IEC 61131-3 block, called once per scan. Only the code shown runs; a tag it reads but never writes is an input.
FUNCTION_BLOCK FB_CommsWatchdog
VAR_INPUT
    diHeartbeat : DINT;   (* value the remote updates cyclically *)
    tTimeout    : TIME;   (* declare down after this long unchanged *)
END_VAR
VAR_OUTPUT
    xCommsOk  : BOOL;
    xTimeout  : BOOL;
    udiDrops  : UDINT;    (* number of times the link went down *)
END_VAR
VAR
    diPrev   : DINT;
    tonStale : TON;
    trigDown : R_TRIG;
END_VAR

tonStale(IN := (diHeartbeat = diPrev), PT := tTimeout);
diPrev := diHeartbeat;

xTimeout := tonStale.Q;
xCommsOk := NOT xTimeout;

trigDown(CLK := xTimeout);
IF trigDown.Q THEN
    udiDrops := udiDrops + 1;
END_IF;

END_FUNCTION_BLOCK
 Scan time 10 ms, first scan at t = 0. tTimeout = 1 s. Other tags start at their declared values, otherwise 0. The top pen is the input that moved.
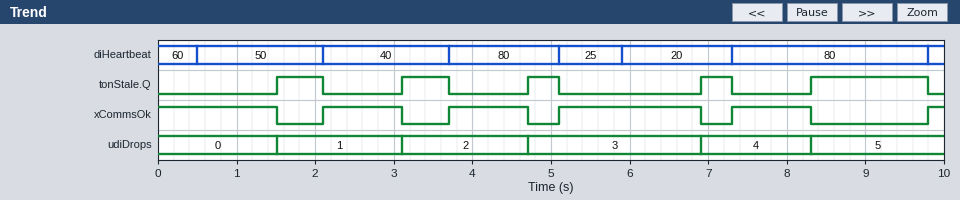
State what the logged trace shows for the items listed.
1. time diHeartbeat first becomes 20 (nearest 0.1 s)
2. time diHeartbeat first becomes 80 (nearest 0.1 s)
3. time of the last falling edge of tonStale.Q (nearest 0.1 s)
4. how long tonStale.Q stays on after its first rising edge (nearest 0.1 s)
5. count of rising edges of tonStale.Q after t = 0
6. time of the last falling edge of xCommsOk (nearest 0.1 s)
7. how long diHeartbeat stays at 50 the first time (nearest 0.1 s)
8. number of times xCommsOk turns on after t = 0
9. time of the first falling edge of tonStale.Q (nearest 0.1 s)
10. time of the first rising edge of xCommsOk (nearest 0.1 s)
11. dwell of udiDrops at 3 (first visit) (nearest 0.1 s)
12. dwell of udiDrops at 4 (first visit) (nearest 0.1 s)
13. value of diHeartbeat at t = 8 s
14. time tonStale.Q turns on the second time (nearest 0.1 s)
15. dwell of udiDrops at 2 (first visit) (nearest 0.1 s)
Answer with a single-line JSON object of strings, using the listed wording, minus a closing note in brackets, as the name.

{"time diHeartbeat first becomes 20": "5.9 s", "time diHeartbeat first becomes 80": "3.7 s", "time of the last falling edge of tonStale.Q": "9.8 s", "how long tonStale.Q stays on after its first rising edge": "0.6 s", "count of rising edges of tonStale.Q after t = 0": "5", "time of the last falling edge of xCommsOk": "8.3 s", "how long diHeartbeat stays at 50 the first time": "1.6 s", "number of times xCommsOk turns on after t = 0": "5", "time of the first falling edge of tonStale.Q": "2.1 s", "time of the first rising edge of xCommsOk": "2.1 s", "dwell of udiDrops at 3 (first visit)": "2.2 s", "dwell of udiDrops at 4 (first visit)": "1.4 s", "value of diHeartbeat at t = 8 s": "80", "time tonStale.Q turns on the second time": "3.1 s", "dwell of udiDrops at 2 (first visit)": "1.6 s"}
